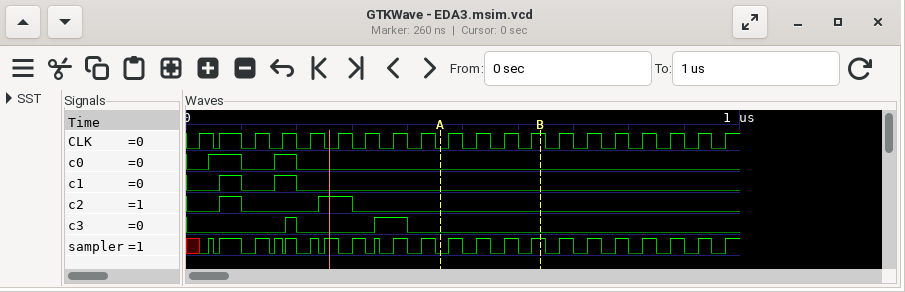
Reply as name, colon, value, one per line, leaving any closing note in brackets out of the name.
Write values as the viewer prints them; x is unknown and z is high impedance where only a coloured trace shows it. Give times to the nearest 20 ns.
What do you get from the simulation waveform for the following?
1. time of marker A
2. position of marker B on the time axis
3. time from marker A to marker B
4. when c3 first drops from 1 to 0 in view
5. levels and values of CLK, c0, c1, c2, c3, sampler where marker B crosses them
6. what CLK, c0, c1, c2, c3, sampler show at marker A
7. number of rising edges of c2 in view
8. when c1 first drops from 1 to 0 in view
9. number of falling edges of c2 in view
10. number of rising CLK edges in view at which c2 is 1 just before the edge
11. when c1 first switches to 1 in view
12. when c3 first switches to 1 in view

time of marker A: 460 ns
position of marker B on the time axis: 640 ns
time from marker A to marker B: 180 ns
when c3 first drops from 1 to 0 in view: 200 ns
levels and values of CLK, c0, c1, c2, c3, sampler where marker B crosses them: CLK=1, c0=0, c1=0, c2=0, c3=0, sampler=1
what CLK, c0, c1, c2, c3, sampler show at marker A: CLK=0, c0=0, c1=0, c2=0, c3=0, sampler=0
number of rising edges of c2 in view: 2
when c1 first drops from 1 to 0 in view: 100 ns
number of falling edges of c2 in view: 2
number of rising CLK edges in view at which c2 is 1 just before the edge: 1
when c1 first switches to 1 in view: 60 ns
when c3 first switches to 1 in view: 180 ns
